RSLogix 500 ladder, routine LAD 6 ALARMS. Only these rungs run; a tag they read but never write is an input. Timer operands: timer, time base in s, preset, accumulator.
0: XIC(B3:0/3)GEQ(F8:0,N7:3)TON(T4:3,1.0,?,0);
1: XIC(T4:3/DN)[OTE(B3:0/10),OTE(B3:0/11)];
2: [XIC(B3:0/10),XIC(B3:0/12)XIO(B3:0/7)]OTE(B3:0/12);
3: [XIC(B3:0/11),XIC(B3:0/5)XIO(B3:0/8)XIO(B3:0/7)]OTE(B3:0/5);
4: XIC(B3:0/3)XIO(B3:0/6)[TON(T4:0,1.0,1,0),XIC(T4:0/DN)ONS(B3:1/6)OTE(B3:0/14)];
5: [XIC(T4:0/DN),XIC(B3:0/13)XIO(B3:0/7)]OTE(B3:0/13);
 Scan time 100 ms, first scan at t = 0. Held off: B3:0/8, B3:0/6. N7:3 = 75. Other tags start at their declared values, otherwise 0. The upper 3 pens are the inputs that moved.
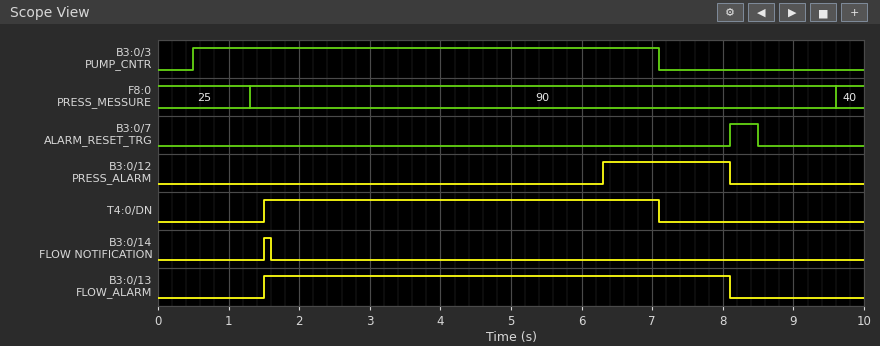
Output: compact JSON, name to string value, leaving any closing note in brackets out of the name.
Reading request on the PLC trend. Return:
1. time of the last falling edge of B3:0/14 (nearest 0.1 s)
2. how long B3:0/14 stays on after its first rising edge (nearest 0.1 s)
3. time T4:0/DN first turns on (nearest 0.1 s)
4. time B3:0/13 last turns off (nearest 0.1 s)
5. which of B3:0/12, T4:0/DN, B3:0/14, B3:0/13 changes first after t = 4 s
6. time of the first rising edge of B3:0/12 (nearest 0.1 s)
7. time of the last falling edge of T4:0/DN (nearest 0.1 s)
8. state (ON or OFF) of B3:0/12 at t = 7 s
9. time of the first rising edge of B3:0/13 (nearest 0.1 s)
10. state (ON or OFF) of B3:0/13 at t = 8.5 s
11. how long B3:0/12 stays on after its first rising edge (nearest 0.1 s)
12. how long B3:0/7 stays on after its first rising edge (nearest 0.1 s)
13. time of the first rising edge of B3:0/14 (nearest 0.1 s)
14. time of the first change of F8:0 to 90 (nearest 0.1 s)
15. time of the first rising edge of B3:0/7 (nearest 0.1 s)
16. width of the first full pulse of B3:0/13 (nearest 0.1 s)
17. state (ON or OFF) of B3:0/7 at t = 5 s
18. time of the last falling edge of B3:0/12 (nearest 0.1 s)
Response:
{"time of the last falling edge of B3:0/14": "1.6 s", "how long B3:0/14 stays on after its first rising edge": "0.1 s", "time T4:0/DN first turns on": "1.5 s", "time B3:0/13 last turns off": "8.1 s", "which of B3:0/12, T4:0/DN, B3:0/14, B3:0/13 changes first after t = 4 s": "B3:0/12", "time of the first rising edge of B3:0/12": "6.3 s", "time of the last falling edge of T4:0/DN": "7.1 s", "state (ON or OFF) of B3:0/12 at t = 7 s": "ON", "time of the first rising edge of B3:0/13": "1.5 s", "state (ON or OFF) of B3:0/13 at t = 8.5 s": "OFF", "how long B3:0/12 stays on after its first rising edge": "1.8 s", "how long B3:0/7 stays on after its first rising edge": "0.4 s", "time of the first rising edge of B3:0/14": "1.5 s", "time of the first change of F8:0 to 90": "1.3 s", "time of the first rising edge of B3:0/7": "8.1 s", "width of the first full pulse of B3:0/13": "6.6 s", "state (ON or OFF) of B3:0/7 at t = 5 s": "OFF", "time of the last falling edge of B3:0/12": "8.1 s"}
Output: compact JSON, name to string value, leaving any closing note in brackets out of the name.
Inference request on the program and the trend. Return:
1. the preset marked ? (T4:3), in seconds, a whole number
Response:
{"the preset marked ? (T4:3), in seconds, a whole number": "5 s"}
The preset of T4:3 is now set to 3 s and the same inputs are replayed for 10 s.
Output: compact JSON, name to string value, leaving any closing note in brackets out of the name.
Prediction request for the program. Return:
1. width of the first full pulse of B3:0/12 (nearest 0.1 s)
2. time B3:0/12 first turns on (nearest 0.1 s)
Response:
{"width of the first full pulse of B3:0/12": "3.8 s", "time B3:0/12 first turns on": "4.3 s"}
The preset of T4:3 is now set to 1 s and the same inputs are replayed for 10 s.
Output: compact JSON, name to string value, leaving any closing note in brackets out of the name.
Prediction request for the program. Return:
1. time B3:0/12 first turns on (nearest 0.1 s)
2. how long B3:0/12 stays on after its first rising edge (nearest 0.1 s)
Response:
{"time B3:0/12 first turns on": "2.3 s", "how long B3:0/12 stays on after its first rising edge": "5.8 s"}
